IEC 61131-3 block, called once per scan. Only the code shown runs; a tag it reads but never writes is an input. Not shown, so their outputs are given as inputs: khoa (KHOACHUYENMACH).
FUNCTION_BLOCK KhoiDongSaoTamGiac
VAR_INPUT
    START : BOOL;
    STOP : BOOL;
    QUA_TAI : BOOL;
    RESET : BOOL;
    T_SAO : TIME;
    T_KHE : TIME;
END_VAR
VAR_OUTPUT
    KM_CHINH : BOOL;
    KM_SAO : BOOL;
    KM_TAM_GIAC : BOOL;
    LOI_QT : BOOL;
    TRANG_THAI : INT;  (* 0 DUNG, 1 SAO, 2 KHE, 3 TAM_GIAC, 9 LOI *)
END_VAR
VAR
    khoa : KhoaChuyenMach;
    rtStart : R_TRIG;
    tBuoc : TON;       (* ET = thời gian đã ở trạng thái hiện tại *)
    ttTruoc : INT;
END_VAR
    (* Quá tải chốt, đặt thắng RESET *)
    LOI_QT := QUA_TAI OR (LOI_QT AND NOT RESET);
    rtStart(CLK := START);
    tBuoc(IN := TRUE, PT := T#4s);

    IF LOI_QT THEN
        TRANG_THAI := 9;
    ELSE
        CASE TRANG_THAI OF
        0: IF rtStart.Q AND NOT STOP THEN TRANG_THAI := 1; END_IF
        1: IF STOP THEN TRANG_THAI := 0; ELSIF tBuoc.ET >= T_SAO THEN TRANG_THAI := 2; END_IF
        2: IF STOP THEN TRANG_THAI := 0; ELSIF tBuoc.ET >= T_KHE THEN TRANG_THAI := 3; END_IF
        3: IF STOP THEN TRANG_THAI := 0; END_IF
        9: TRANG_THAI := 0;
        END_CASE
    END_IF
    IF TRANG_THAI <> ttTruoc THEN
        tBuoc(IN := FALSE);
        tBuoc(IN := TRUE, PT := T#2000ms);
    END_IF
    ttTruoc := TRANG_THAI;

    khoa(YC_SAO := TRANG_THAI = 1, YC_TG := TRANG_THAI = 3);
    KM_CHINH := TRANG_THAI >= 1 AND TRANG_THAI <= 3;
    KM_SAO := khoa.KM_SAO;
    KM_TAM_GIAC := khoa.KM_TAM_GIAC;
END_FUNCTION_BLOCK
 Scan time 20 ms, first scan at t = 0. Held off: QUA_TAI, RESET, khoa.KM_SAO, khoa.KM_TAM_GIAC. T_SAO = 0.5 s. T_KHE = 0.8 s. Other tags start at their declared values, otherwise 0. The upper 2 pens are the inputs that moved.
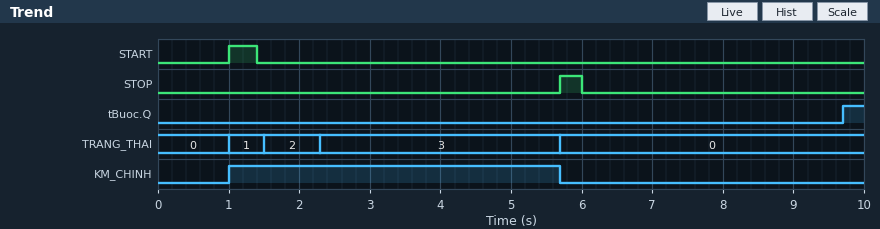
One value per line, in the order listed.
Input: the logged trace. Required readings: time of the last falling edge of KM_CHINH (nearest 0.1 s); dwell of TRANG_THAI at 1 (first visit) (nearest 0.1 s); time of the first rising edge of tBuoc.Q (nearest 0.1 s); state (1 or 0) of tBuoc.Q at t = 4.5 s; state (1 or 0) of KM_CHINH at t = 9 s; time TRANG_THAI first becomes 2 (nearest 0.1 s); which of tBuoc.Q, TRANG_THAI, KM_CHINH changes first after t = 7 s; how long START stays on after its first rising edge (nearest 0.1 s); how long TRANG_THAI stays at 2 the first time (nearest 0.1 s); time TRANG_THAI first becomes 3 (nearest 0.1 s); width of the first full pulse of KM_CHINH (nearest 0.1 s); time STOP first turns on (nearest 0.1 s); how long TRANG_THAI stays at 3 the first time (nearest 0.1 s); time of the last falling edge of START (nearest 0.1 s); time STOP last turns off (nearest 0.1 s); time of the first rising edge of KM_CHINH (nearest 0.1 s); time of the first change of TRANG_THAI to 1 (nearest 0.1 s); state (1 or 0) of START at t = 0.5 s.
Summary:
5.7 s
0.5 s
9.7 s
0
0
1.5 s
tBuoc.Q
0.4 s
0.8 s
2.3 s
4.7 s
5.7 s
3.4 s
1.4 s
6.0 s
1.0 s
1.0 s
0
